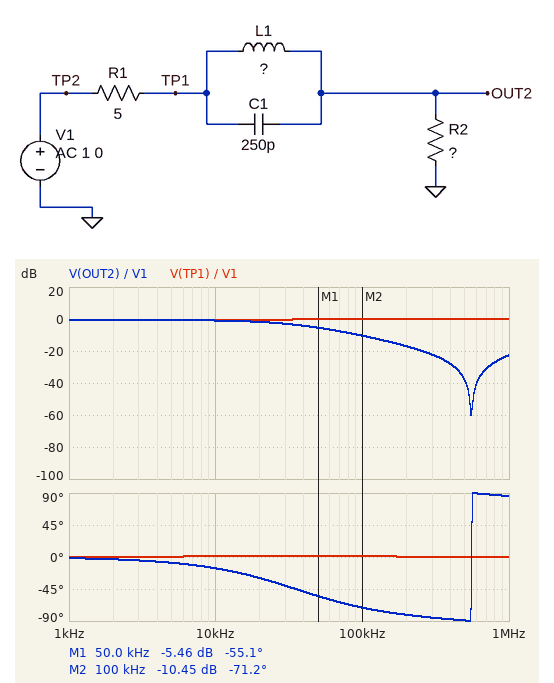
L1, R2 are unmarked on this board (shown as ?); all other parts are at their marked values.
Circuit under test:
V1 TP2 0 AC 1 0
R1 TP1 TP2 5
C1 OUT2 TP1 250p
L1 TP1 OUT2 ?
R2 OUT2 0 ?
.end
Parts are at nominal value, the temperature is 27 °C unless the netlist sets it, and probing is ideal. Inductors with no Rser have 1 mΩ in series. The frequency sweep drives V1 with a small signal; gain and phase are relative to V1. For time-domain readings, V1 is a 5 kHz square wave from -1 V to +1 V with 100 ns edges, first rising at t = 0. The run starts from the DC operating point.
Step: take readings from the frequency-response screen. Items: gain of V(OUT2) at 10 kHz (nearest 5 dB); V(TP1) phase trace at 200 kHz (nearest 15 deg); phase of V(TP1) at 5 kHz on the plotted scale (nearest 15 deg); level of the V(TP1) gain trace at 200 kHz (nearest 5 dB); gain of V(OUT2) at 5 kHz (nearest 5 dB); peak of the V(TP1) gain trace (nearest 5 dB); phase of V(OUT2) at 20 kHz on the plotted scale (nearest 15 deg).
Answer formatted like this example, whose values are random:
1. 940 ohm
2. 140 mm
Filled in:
1. 0 dB
2. 0 deg
3. 0 deg
4. 0 dB
5. 0 dB
6. 0 dB
7. -30 deg
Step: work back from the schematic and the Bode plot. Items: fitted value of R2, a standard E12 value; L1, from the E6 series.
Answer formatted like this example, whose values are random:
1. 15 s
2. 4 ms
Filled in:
1. 68 Ω
2. 330 µH
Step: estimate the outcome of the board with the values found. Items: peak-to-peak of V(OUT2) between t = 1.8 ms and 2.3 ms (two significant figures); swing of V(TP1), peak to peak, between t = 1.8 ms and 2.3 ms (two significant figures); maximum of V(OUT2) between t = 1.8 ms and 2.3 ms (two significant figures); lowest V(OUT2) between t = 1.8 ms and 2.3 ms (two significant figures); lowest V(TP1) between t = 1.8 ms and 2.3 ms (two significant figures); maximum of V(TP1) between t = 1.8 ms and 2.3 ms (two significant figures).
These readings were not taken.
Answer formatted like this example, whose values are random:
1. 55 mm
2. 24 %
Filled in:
1. 1.9 V
2. 2.1 V
3. 930 mV
4. -930 mV
5. -1.1 V
6. 1.1 V
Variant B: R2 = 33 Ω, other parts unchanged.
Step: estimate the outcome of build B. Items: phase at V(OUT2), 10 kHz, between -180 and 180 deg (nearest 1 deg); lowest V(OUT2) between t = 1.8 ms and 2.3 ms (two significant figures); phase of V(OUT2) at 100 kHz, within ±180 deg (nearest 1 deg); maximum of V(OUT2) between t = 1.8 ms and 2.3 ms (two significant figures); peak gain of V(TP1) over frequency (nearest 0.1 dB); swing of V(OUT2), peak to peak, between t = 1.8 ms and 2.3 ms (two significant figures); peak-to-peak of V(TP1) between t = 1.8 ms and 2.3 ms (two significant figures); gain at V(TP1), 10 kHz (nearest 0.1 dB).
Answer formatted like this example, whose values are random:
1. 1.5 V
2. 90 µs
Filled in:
1. -29 deg
2. -870 mV
3. -80 deg
4. 870 mV
5. 0 dB
6. 1.7 V
7. 2.3 V
8. -0.9 dB
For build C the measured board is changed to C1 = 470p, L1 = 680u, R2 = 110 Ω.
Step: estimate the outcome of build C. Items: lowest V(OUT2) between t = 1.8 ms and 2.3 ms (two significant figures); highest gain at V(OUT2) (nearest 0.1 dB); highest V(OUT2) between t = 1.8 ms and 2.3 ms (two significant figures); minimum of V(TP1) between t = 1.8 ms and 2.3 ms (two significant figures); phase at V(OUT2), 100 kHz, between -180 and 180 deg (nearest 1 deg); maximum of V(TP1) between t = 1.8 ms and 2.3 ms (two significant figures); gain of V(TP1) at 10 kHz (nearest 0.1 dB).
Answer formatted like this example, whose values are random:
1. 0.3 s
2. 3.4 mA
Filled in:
1. -960 mV
2. -0.4 dB
3. 960 mV
4. -1.0 V
5. -77 deg
6. 1.0 V
7. -0.3 dB
